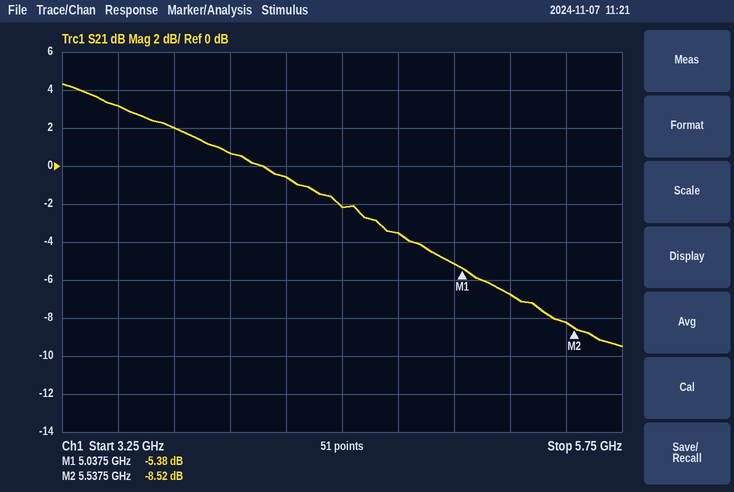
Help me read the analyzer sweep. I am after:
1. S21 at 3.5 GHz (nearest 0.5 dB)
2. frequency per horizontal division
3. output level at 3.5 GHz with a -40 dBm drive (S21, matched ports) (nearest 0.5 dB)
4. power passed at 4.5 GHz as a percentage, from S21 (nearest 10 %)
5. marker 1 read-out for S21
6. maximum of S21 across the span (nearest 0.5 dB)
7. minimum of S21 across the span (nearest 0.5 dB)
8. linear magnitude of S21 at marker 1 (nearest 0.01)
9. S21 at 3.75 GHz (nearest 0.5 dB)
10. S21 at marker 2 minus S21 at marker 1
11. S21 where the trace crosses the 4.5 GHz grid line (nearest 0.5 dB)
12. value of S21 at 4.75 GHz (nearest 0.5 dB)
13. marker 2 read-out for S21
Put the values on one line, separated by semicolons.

3.0 dB; 250 MHz; -37.0 dBm; 60 %; -5.38 dB; 4.5 dB; -9.5 dB; 0.54; 2.0 dB; -3.14 dB; -2.0 dB; -3.5 dB; -8.52 dB
